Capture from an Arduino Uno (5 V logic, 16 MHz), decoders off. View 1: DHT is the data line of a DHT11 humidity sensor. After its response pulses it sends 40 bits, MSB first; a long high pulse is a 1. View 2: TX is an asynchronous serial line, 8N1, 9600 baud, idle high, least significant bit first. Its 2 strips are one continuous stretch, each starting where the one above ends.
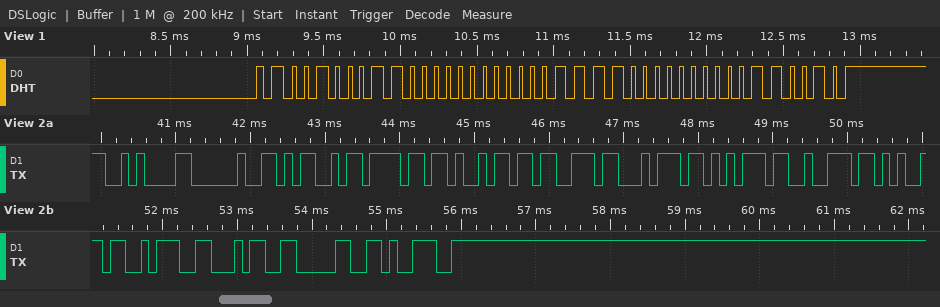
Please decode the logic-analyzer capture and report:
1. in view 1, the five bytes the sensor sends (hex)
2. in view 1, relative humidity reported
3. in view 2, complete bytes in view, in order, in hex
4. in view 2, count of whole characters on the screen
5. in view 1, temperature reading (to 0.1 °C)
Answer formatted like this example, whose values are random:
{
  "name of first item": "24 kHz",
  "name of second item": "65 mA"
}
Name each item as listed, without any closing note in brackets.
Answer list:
{
  "in view 1, the five bytes the sensor sends": "23 00 0F 00 32",
  "in view 1, relative humidity reported": "35 %",
  "in view 2, complete bytes in view, in order, in hex": "0A 20 4D 6F 69 73 74 75 72 65 3A 34 30 39",
  "in view 2, count of whole characters on the screen": "14",
  "in view 1, temperature reading": "15.0 °C"
}
